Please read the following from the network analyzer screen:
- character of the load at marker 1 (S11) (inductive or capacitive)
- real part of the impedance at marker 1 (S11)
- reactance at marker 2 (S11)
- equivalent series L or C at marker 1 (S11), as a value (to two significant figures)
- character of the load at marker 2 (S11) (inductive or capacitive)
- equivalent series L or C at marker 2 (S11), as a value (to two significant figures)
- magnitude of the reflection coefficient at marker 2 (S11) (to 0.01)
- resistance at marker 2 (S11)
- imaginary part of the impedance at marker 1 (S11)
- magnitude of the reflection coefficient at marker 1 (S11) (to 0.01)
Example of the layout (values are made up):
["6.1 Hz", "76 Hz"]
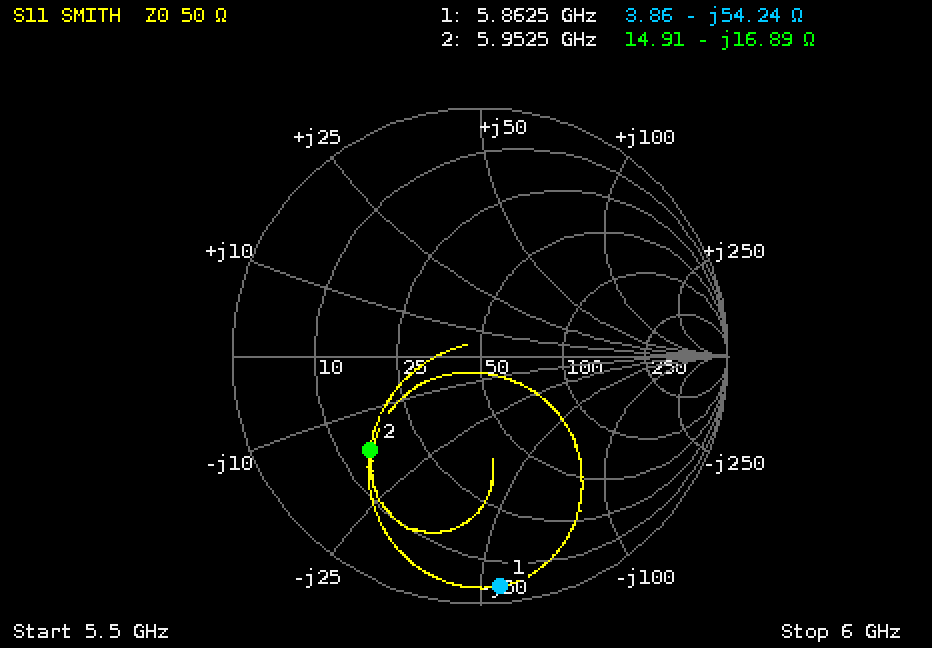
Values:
["capacitive", "3.86 Ω", "-16.89 Ω", "500 fF", "capacitive", "1.6 pF", "0.58", "14.91 Ω", "-54.24 Ω", "0.93"]
